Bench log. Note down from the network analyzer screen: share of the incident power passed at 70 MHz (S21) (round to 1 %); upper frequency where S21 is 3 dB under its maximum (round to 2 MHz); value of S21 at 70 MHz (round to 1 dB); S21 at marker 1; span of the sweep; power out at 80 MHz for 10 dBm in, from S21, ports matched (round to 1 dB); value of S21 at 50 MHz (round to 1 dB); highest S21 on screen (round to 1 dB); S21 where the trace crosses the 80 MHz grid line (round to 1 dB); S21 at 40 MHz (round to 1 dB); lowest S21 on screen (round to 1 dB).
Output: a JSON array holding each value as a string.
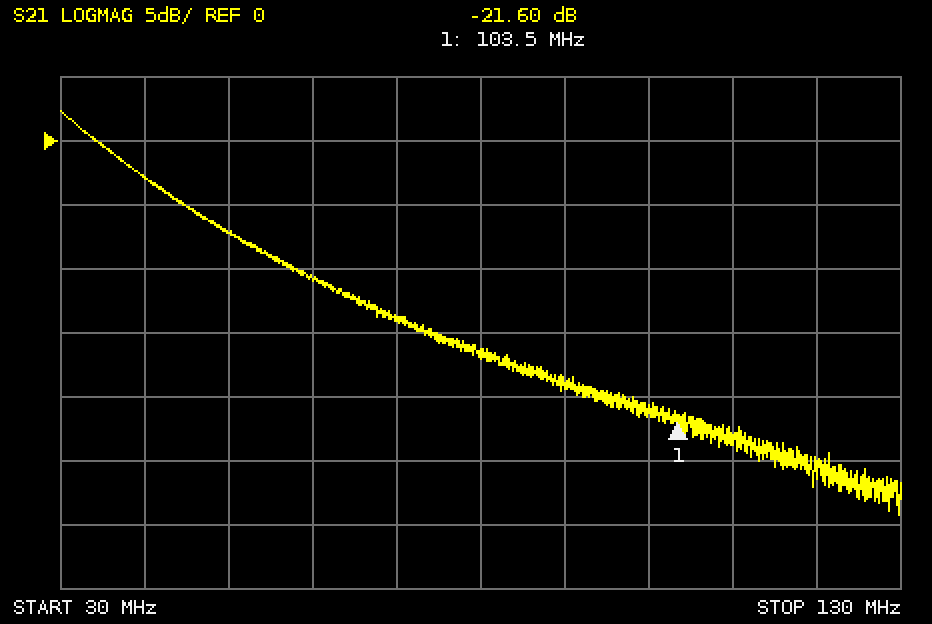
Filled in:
["4 %", "36 MHz", "-14 dB", "-21.60 dB", "100 MHz", "-7 dBm", "-7 dB", "2 dB", "-17 dB", "-3 dB", "-29 dB"]
